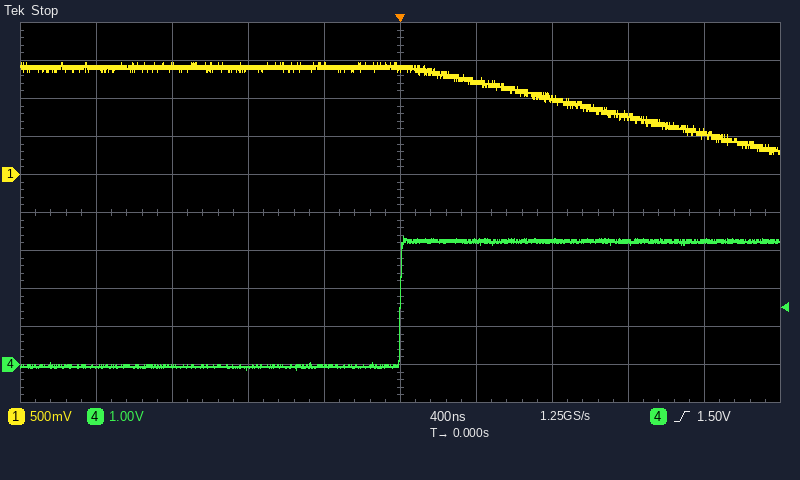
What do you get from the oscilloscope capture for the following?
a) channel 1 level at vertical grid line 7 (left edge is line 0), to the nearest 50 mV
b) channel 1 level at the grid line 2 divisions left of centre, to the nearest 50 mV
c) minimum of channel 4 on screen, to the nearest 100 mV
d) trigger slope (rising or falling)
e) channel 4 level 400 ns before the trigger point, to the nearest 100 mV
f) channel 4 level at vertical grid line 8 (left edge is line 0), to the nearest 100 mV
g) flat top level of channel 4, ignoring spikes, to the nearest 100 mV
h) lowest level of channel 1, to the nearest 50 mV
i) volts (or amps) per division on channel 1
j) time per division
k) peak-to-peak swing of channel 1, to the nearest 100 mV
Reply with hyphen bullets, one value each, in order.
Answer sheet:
- 1.00 V
- 1.40 V
- -100 mV
- rising
- 0.0 V
- 3.2 V
- 3.2 V
- 300 mV
- 500 mV
- 400 ns
- 1.20 V
